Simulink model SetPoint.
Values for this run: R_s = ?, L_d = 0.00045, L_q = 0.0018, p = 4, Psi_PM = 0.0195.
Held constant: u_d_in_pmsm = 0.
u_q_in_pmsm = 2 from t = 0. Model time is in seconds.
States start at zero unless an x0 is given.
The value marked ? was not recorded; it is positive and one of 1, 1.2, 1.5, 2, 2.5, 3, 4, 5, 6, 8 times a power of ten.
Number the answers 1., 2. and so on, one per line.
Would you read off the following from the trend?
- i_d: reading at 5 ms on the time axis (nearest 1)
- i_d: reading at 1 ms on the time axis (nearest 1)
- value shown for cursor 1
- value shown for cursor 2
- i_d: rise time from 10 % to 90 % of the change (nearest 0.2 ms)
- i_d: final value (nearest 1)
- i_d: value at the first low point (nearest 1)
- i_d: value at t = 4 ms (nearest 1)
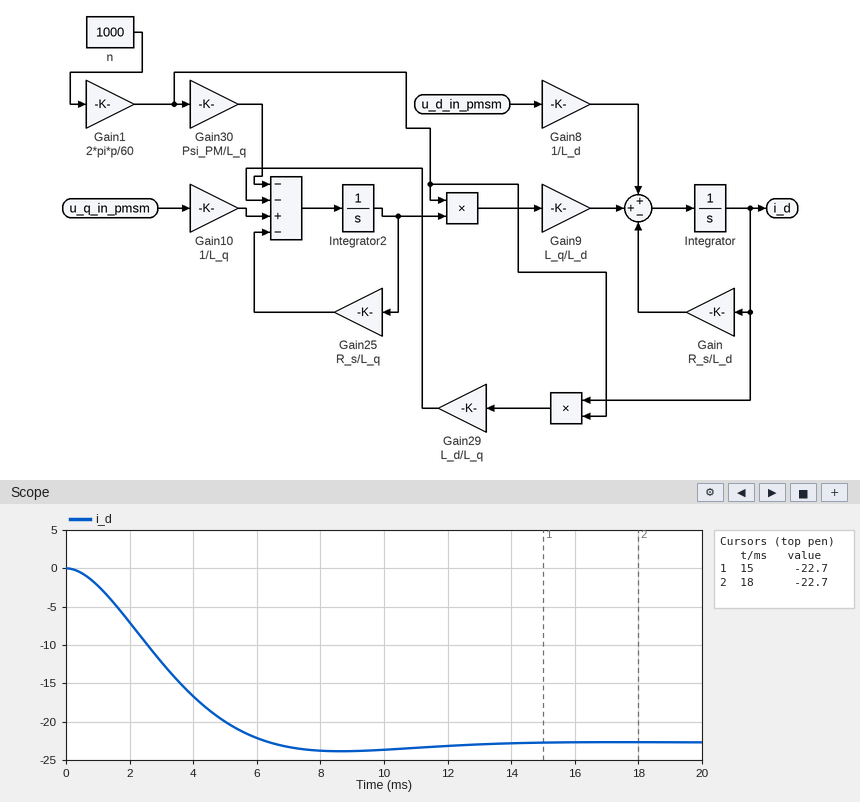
1. -20
2. -2
3. -22.7
4. -22.7
5. 4.2 ms
6. -23
7. -24
8. -17
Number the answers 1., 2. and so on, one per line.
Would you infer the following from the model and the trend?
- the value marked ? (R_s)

1. 0.25
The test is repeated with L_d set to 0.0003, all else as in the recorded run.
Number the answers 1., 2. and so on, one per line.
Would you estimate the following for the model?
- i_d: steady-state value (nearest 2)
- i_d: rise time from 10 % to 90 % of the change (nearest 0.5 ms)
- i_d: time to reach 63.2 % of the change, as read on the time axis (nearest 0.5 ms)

1. -30
2. 5.5 ms
3. 3.5 ms
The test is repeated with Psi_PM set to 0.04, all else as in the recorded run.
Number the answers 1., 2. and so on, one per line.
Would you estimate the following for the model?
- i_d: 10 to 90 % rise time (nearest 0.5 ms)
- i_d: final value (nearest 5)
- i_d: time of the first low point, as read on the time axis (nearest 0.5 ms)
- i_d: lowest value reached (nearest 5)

1. 4.0 ms
2. -55
3. 8.5 ms
4. -55
